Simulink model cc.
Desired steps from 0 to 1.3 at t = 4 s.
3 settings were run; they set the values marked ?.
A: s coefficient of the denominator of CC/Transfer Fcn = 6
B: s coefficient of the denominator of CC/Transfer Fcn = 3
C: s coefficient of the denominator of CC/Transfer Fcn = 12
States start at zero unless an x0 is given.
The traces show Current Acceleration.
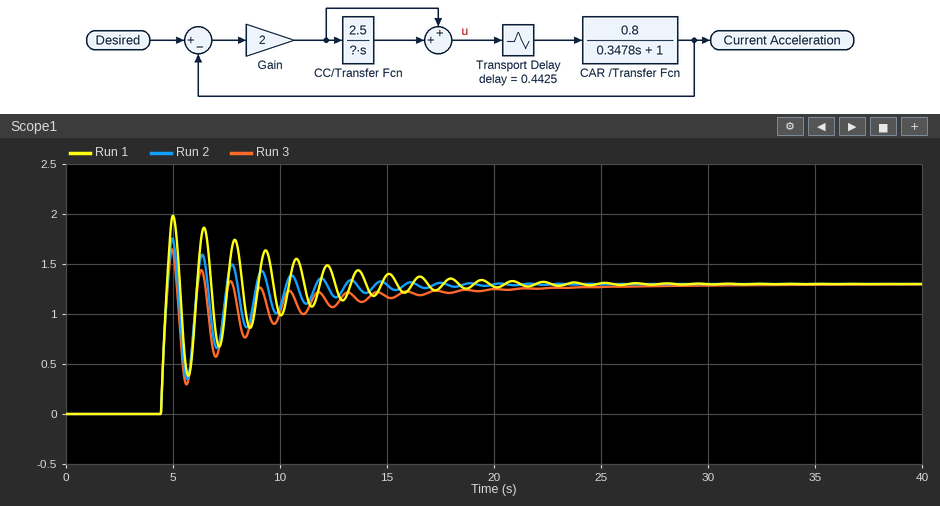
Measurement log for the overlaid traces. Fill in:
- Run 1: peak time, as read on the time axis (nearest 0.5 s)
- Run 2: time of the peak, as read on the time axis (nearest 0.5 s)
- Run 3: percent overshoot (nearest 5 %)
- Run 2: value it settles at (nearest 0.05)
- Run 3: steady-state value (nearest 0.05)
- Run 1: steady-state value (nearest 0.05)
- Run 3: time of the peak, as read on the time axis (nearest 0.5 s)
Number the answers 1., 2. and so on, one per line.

1. 5.0 s
2. 5.0 s
3. 25 %
4. 1.30
5. 1.30
6. 1.30
7. 5.0 s
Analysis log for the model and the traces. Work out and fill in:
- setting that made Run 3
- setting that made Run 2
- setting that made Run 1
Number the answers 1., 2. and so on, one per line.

1. C
2. A
3. B
